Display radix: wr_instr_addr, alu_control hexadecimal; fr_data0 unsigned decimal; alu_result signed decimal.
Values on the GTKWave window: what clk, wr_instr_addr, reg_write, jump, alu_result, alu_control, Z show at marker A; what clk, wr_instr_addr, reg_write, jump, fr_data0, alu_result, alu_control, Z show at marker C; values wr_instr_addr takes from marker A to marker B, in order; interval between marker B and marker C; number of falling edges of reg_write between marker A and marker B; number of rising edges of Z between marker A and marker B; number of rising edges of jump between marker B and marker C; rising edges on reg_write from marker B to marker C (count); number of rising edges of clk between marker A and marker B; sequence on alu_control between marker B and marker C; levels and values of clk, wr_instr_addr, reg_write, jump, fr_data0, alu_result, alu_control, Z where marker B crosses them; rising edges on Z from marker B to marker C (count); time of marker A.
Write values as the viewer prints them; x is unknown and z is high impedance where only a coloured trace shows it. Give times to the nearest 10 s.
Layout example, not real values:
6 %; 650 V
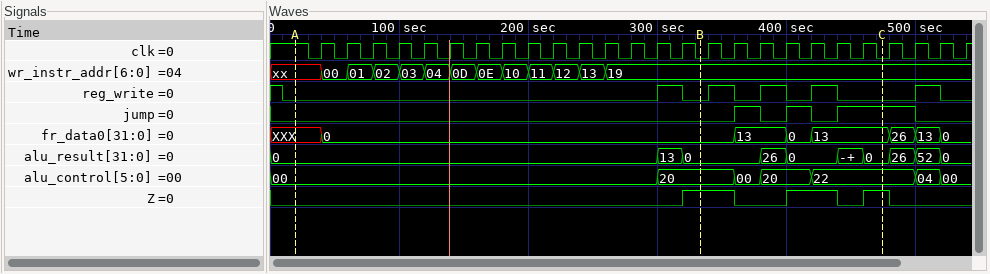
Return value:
clk=1, wr_instr_addr=xx, reg_write=0, jump=0, alu_result=0, alu_control=00, Z=0; clk=0, wr_instr_addr=19, reg_write=0, jump=1, fr_data0=13, alu_result=0, alu_control=22, Z=1; xx, 00, 01, 02, 03, 04, 0D, 0E, 10, 11, 12, 13, 19; 140 s; 1; 1; 3; 3; 15; 20, 00, 20, 22; clk=0, wr_instr_addr=19, reg_write=0, jump=0, fr_data0=0, alu_result=0, alu_control=20, Z=1; 2; 20 s
